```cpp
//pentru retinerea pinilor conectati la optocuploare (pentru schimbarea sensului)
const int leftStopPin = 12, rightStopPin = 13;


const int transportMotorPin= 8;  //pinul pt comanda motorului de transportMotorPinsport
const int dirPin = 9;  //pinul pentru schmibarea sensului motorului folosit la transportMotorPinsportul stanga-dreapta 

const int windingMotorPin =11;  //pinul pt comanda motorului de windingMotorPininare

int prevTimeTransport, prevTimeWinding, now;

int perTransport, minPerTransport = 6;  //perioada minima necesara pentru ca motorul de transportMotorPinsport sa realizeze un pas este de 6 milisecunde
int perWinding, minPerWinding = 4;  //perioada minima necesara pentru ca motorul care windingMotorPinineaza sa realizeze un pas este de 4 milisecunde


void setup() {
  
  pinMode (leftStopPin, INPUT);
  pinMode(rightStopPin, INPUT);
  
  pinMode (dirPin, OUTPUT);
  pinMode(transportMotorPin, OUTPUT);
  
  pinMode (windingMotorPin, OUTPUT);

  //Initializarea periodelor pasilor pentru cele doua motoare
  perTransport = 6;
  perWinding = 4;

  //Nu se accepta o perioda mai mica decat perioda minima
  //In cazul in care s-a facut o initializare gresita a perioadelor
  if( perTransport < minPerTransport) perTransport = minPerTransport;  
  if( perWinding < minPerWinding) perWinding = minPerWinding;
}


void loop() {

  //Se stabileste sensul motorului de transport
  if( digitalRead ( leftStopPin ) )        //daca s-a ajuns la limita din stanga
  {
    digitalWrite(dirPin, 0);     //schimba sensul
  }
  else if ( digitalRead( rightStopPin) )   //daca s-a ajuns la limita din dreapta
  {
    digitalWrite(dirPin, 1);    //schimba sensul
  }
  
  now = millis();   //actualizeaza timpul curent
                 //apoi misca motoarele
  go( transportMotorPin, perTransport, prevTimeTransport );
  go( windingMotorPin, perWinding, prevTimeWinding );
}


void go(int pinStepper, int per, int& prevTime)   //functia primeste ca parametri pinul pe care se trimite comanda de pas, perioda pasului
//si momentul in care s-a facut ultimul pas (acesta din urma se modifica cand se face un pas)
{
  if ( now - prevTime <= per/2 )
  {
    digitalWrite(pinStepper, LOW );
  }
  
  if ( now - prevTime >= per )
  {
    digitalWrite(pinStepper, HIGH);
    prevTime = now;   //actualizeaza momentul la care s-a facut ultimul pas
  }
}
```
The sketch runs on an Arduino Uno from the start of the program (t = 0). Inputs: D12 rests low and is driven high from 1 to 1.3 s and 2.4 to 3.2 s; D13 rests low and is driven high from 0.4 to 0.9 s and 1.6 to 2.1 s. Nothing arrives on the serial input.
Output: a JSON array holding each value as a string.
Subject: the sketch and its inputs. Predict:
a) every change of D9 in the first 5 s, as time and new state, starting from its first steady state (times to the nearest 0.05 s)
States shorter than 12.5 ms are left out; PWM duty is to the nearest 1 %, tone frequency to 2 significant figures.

["0 s low; 0.4 s high; 1 s low; 1.6 s high; 2.4 s low"]
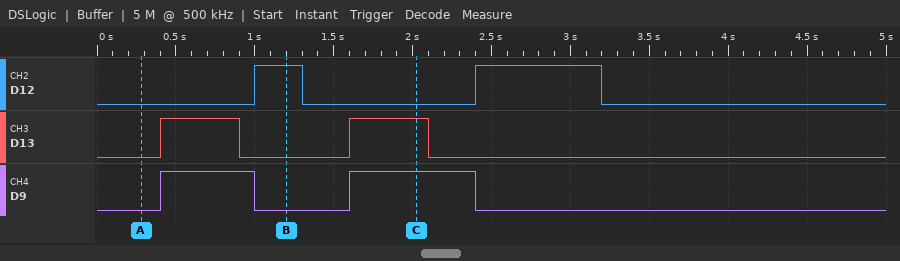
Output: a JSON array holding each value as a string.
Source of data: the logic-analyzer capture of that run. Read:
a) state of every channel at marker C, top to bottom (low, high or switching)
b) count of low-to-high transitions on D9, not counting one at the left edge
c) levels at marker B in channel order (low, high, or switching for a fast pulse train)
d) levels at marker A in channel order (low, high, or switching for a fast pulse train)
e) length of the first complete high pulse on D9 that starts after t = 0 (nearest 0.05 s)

["D12 low, D13 high, D9 high", "2", "D12 high, D13 low, D9 low", "D12 low, D13 low, D9 low", "0.60 s"]
